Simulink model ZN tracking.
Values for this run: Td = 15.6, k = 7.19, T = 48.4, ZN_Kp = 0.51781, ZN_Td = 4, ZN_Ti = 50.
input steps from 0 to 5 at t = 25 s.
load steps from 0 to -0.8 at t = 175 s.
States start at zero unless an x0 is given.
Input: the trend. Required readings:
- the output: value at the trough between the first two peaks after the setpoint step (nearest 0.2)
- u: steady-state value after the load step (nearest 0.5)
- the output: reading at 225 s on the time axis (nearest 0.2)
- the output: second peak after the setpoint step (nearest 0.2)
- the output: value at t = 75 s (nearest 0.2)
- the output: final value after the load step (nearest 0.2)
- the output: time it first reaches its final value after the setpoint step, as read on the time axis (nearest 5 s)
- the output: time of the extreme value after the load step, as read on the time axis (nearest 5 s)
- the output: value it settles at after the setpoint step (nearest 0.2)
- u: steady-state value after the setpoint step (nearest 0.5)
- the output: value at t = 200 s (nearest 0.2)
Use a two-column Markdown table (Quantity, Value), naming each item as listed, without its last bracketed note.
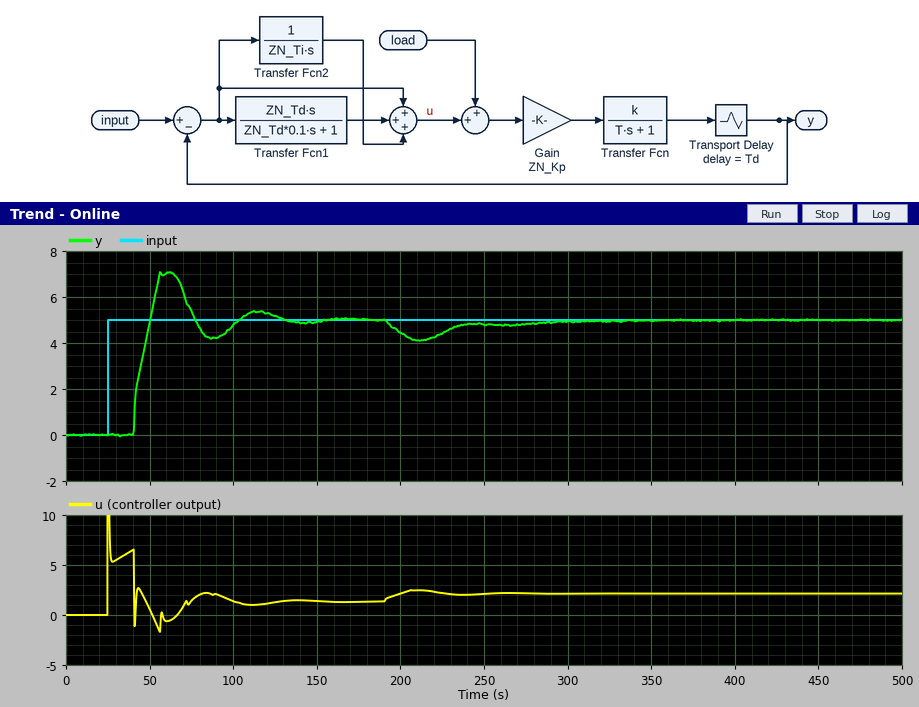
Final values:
| Quantity | Value |
|---|---|
| the output: value at the trough between the first two peaks after the setpoint step | 4.2 |
| u: steady-state value after the load step | 2.0 |
| the output: reading at 225 s on the time axis | 4.4 |
| the output: second peak after the setpoint step | 5.4 |
| the output: value at t = 75 s | 5.4 |
| the output: final value after the load step | 5.0 |
| the output: time it first reaches its final value after the setpoint step, as read on the time axis | 50 s |
| the output: time of the extreme value after the load step, as read on the time axis | 210 s |
| the output: value it settles at after the setpoint step | 5.0 |
| u: steady-state value after the setpoint step | 1.5 |
| the output: value at t = 200 s | 4.4 |
